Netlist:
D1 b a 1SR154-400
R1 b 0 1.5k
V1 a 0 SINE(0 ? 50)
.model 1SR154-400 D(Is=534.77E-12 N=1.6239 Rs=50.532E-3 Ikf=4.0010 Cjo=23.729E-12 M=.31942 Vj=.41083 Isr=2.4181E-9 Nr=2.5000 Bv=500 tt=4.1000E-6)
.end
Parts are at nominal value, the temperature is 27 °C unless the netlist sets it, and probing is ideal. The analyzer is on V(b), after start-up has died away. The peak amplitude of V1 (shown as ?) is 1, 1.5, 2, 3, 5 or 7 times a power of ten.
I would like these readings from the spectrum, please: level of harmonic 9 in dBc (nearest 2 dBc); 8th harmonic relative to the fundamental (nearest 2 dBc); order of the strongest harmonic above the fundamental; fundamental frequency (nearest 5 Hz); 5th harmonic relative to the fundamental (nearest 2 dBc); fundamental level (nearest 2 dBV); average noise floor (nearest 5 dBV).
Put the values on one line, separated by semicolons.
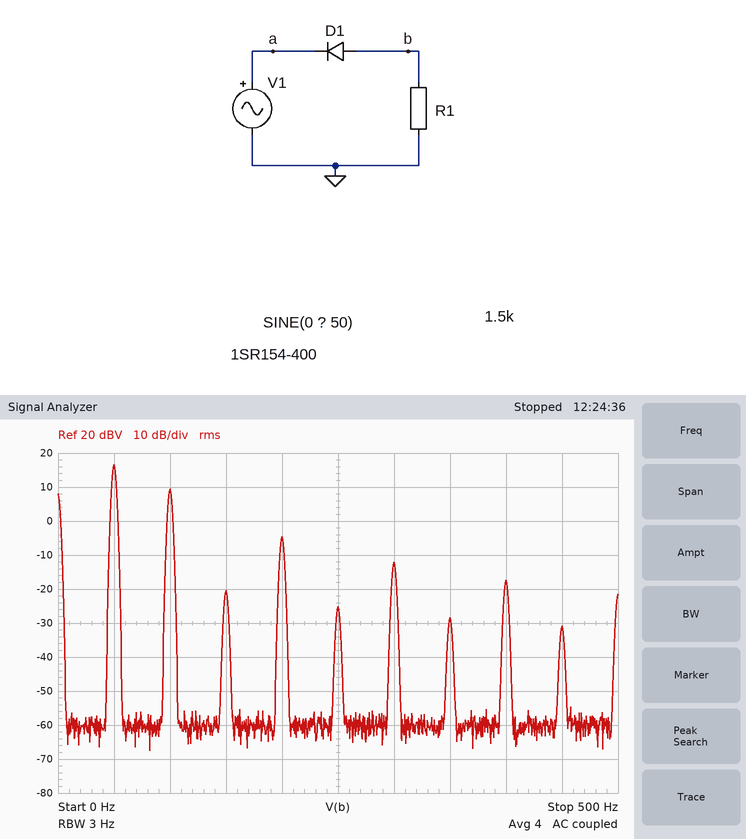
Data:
-48 dBc; -34 dBc; 2; 50 Hz; -42 dBc; 16 dBV; -60 dBV
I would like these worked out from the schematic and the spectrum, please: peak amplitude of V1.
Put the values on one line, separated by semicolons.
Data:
20 V
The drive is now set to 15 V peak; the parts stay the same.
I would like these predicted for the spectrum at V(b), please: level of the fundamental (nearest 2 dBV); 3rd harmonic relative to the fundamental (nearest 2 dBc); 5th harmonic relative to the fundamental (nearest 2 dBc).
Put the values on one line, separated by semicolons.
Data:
14 dBV; -34 dBc; -40 dBc
